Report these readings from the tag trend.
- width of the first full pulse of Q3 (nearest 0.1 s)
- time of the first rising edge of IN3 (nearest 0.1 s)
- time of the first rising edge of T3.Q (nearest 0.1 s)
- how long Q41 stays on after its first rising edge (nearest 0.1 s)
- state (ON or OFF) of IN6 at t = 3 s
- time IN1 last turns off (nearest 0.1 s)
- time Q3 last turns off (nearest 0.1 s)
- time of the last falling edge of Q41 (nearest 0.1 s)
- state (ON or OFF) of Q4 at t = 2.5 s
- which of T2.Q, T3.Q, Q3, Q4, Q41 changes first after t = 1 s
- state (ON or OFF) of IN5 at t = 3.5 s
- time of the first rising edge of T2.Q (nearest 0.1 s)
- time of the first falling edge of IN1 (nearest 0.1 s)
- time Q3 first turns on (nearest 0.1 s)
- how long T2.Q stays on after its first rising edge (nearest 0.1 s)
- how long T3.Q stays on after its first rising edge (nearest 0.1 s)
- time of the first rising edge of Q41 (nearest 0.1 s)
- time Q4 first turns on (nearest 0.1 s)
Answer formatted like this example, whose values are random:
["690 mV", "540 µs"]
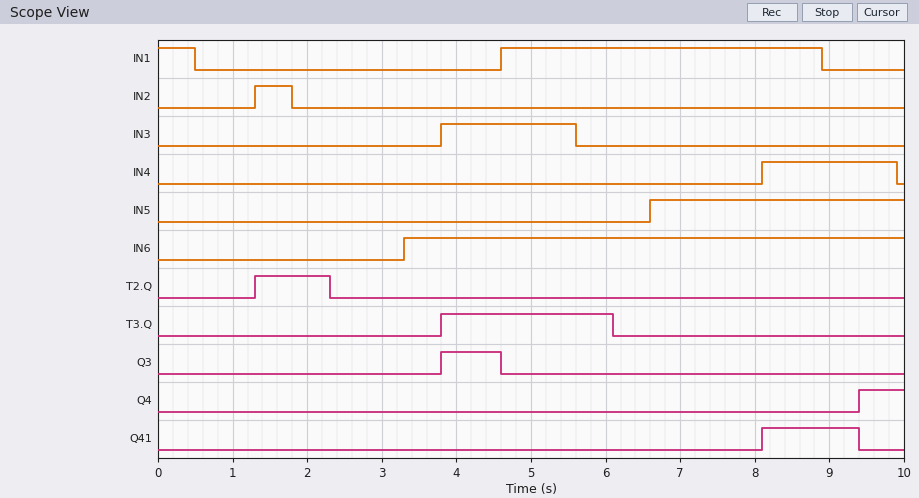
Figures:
["0.8 s", "3.8 s", "3.8 s", "1.3 s", "OFF", "8.9 s", "4.6 s", "9.4 s", "OFF", "T2.Q", "OFF", "1.3 s", "0.5 s", "3.8 s", "1.0 s", "2.3 s", "8.1 s", "9.4 s"]
